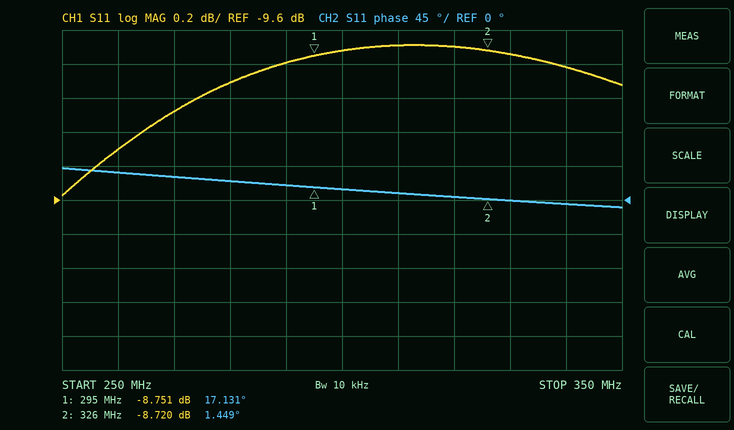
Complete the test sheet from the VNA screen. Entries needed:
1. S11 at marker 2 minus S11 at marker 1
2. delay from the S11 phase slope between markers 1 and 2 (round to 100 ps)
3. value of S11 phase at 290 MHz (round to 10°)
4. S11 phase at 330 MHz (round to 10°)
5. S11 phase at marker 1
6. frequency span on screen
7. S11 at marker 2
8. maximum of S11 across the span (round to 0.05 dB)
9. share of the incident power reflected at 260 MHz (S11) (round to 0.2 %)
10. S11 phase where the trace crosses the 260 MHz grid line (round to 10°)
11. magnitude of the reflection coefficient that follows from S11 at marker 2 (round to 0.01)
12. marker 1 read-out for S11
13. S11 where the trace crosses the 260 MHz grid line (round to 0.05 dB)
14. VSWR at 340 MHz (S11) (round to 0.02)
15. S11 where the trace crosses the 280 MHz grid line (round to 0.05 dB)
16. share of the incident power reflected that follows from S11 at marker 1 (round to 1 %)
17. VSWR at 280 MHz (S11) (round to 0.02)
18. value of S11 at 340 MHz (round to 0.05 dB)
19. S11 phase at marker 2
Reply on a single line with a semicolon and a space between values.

0.031 dB; 1.4 ns; 20°; 0°; 17.131°; 100 MHz; -8.720 dB; -8.70 dB; 11.8 %; 40°; 0.37; -8.751 dB; -9.30 dB; 2.14; -8.90 dB; 13 %; 2.12; -8.80 dB; 1.449°
